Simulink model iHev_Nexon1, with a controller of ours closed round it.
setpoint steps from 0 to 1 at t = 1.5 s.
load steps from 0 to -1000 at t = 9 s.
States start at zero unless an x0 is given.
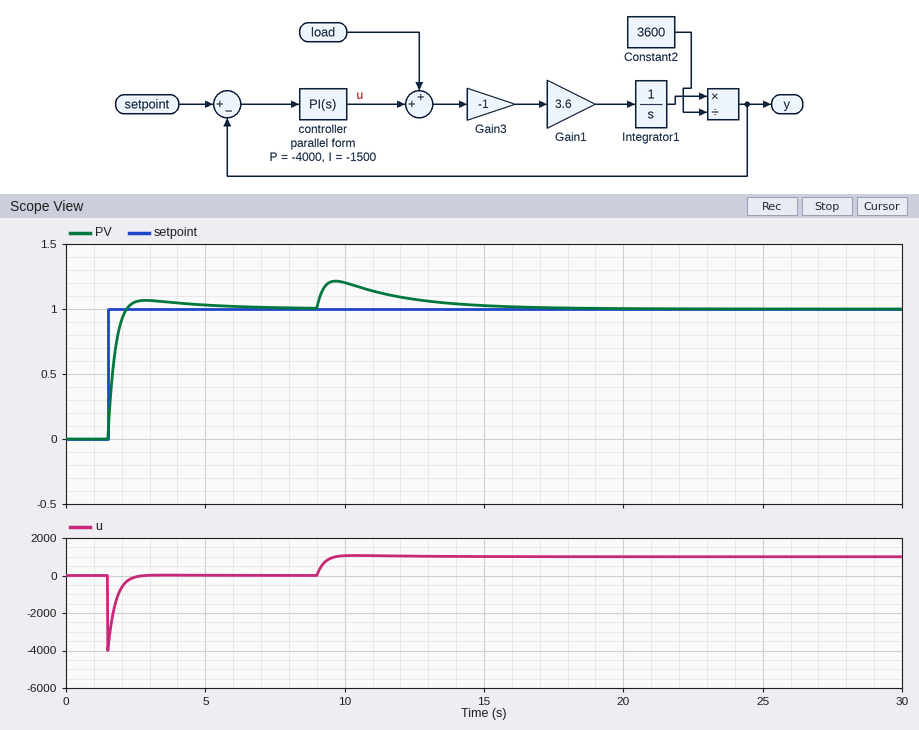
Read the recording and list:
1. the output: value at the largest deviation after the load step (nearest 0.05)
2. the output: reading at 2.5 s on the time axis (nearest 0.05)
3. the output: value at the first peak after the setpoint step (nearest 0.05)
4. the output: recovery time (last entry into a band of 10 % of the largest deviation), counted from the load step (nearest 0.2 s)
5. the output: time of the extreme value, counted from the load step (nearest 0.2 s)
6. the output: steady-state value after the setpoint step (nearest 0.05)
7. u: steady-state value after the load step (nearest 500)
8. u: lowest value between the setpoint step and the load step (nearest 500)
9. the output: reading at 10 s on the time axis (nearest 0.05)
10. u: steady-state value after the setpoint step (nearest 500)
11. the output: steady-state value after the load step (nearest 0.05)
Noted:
1.20
1.05
1.05
6.6 s
0.6 s
1.00
1000
-4000
1.20
0
1.00
